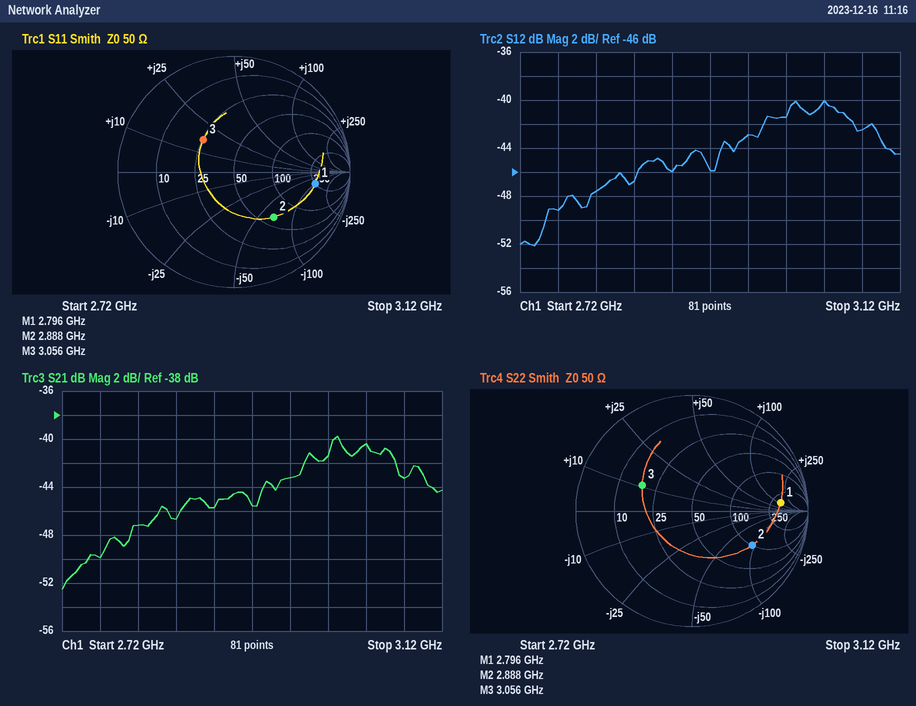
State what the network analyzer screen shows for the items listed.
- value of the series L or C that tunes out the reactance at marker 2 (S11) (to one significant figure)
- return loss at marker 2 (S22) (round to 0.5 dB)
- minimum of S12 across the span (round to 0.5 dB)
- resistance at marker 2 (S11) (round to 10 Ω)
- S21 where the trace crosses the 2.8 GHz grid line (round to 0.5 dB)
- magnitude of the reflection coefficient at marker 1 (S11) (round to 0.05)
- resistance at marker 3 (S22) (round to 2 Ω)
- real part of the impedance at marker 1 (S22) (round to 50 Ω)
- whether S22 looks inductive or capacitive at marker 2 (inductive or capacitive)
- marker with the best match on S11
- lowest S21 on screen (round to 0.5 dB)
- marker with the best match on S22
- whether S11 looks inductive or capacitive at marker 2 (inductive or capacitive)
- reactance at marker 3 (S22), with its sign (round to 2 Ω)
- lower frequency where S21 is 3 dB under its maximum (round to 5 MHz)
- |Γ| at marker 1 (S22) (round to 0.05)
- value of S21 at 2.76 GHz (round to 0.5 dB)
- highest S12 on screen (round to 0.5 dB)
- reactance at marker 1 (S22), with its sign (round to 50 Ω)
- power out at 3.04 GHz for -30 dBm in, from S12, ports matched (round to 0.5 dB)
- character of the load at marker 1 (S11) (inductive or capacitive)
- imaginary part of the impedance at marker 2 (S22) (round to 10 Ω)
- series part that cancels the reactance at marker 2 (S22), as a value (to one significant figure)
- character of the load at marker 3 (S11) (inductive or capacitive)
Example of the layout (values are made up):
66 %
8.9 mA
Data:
4 nH
4.5 dB
-52.0 dB
60 Ω
-47.0 dB
0.70
18 Ω
350 Ω
capacitive
marker 3
-52.5 dB
marker 3
capacitive
+10 Ω
2.970 GHz
0.75
-50.0 dB
-40.0 dB
+100 Ω
-70.0 dBm
capacitive
-90 Ω
5 nH
inductive
